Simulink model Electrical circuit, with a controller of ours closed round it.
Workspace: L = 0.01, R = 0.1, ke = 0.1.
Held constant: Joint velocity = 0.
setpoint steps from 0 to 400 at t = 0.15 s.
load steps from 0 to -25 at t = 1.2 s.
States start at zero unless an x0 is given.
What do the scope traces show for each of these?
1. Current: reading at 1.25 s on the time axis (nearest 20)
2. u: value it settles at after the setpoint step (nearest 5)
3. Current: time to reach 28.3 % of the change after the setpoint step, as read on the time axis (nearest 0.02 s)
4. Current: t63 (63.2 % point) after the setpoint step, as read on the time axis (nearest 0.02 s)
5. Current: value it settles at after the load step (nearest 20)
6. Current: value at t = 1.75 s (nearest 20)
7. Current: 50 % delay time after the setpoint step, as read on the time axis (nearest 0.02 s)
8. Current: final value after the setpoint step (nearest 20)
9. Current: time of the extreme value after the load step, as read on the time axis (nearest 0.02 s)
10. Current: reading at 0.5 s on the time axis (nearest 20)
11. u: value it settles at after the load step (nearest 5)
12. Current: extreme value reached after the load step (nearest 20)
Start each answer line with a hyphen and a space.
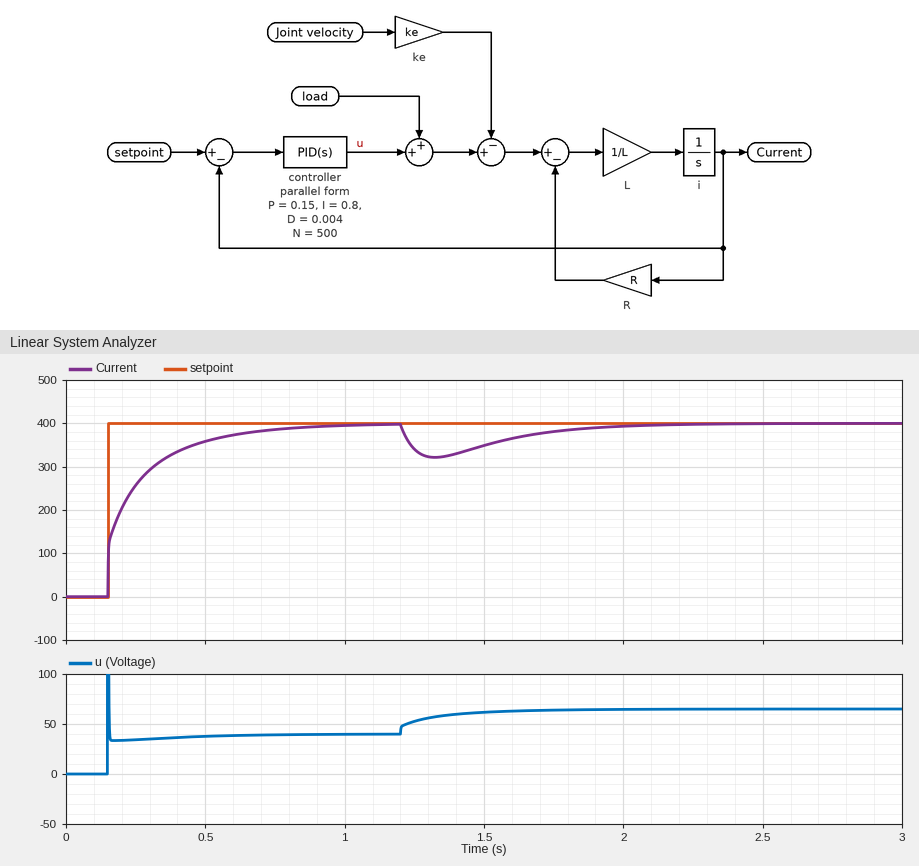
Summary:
- 340
- 40
- 0.16 s
- 0.24 s
- 400
- 380
- 0.20 s
- 400
- 1.32 s
- 360
- 65
- 320
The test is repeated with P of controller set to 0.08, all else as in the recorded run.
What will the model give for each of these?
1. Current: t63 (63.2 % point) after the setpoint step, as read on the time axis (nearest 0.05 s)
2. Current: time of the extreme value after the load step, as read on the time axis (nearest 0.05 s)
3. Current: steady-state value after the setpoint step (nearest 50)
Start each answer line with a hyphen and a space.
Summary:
- 0.30 s
- 1.35 s
- 400
